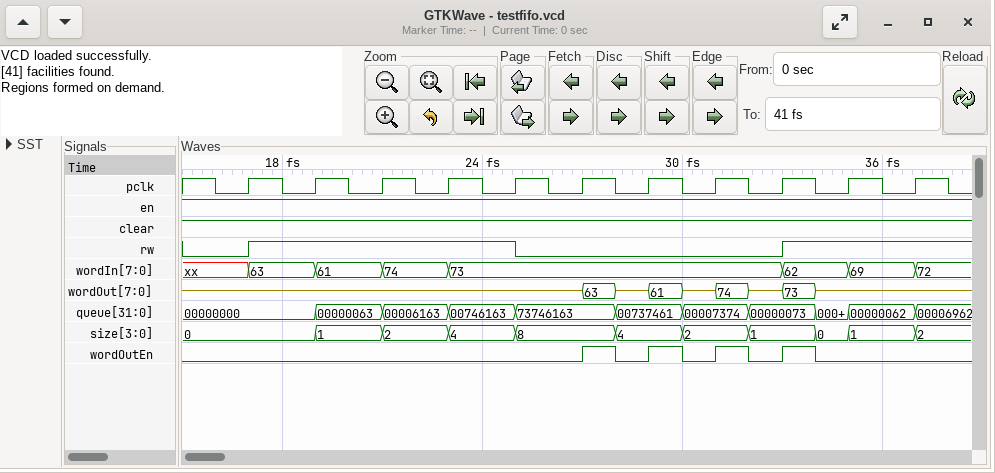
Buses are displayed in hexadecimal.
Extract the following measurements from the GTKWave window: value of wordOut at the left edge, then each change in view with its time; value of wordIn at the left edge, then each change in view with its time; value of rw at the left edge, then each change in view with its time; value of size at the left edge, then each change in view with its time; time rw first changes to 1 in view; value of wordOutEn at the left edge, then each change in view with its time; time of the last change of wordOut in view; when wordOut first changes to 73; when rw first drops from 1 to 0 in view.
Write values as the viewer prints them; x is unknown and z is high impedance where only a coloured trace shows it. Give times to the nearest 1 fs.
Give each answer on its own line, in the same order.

z, 63 at 27 fs, z at 28 fs, 61 at 29 fs, z at 30 fs, 74 at 31 fs, z at 32 fs, 73 at 33 fs, z at 34 fs
xx, 63 at 17 fs, 61 at 19 fs, 74 at 21 fs, 73 at 23 fs, 62 at 33 fs, 69 at 35 fs, 72 at 37 fs
0, 1 at 17 fs, 0 at 25 fs, 1 at 33 fs
0, 1 at 19 fs, 2 at 21 fs, 4 at 23 fs, 8 at 25 fs, 4 at 28 fs, 2 at 30 fs, 1 at 32 fs, 0 at 34 fs, 1 at 35 fs, 2 at 37 fs
17 fs
0, 1 at 27 fs, 0 at 28 fs, 1 at 29 fs, 0 at 30 fs, 1 at 31 fs, 0 at 32 fs, 1 at 33 fs, 0 at 34 fs
34 fs
33 fs
25 fs
